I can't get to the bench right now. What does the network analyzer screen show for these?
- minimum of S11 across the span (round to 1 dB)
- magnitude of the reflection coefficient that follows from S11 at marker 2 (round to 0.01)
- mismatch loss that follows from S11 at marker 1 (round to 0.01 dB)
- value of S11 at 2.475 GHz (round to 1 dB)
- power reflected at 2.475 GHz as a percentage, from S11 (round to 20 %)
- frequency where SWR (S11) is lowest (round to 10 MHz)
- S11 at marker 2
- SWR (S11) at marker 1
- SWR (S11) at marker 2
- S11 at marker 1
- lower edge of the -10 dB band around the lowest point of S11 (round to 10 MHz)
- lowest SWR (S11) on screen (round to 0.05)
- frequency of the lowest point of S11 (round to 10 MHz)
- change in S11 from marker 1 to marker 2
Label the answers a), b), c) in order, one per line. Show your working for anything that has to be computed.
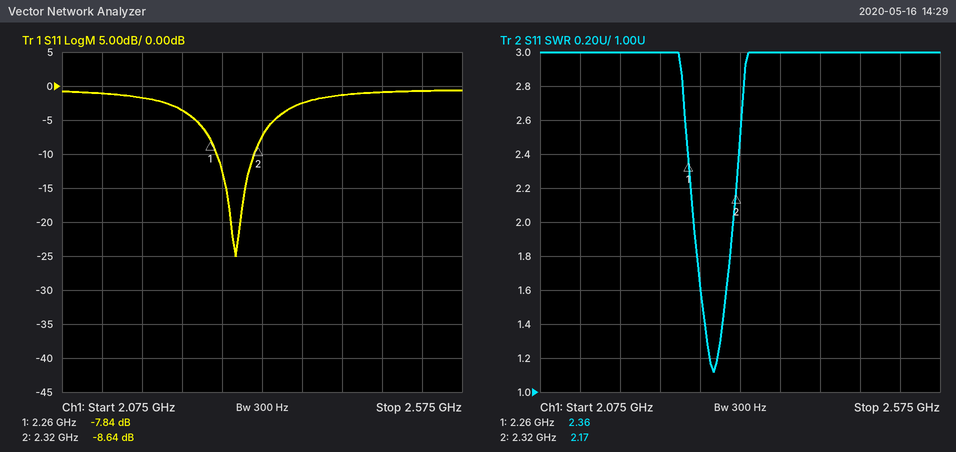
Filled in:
a) -25 dB
b) 10^(-8.64/20) ≈ 0.37
c) −10 log10(1 − 10^(-7.84/10)) ≈ 0.78 dB
d) -1 dB
e) 10^(-1/10) ≈ 79.4 %, so 80 % to the nearest 20 %
f) 2.29 GHz
g) -8.64 dB
h) 2.36
i) 2.17
j) -7.84 dB
k) 2.27 GHz
l) 1.10
m) 2.29 GHz
n) -8.64 − (-7.84) = -0.80 dB
